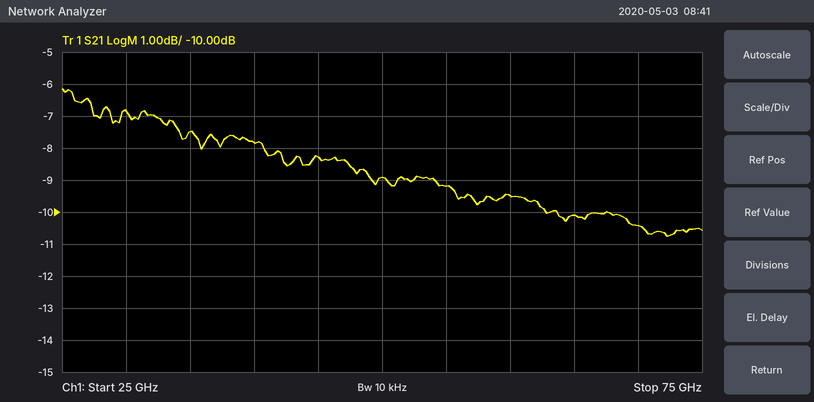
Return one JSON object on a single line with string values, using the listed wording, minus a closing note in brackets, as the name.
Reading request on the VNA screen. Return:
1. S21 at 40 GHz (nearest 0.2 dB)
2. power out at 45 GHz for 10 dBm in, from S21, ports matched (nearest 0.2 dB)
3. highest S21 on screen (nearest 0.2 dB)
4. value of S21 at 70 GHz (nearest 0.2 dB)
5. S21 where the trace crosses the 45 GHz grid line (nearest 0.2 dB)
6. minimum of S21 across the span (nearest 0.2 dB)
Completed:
{"S21 at 40 GHz": "-7.8 dB", "power out at 45 GHz for 10 dBm in, from S21, ports matched": "1.8 dBm", "highest S21 on screen": "-6.2 dB", "value of S21 at 70 GHz": "-10.4 dB", "S21 where the trace crosses the 45 GHz grid line": "-8.2 dB", "minimum of S21 across the span": "-10.8 dB"}
